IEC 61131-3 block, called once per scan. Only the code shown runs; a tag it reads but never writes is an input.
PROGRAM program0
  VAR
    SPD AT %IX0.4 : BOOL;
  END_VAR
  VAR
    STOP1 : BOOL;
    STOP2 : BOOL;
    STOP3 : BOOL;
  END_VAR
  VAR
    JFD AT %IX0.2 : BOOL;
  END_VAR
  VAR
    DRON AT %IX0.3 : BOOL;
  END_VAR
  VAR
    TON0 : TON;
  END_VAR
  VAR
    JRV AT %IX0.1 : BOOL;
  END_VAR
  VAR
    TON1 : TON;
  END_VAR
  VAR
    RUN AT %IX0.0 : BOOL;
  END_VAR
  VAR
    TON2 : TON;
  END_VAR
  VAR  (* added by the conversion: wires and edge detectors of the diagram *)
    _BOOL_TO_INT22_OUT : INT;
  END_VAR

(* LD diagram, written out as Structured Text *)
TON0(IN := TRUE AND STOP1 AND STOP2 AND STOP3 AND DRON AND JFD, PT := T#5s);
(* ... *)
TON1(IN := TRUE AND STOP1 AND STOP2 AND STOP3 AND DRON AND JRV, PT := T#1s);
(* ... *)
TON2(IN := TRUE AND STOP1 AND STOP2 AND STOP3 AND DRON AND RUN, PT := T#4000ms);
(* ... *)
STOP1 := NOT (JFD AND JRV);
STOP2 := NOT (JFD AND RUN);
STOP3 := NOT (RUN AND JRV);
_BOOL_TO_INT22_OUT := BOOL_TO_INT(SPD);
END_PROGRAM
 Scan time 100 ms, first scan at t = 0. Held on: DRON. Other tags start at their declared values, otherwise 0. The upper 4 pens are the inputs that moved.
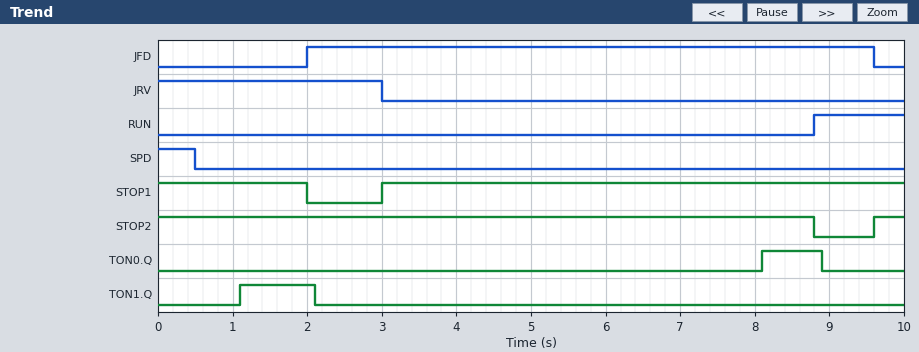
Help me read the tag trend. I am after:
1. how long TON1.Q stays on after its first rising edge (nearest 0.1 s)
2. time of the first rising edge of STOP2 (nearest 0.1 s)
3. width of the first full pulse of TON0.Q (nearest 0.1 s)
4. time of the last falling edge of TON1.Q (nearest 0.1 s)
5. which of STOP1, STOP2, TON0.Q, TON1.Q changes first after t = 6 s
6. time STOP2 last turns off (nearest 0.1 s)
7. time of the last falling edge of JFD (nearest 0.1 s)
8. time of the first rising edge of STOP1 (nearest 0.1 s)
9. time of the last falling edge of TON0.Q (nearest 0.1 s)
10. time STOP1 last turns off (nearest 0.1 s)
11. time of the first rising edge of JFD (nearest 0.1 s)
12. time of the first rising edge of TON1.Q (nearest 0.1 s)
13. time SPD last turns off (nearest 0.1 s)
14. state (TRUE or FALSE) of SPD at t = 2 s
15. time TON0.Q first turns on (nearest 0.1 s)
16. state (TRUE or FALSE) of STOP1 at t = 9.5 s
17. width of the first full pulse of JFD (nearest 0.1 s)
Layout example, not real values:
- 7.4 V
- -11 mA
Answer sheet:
- 1.0 s
- 9.6 s
- 0.8 s
- 2.1 s
- TON0.Q
- 8.8 s
- 9.6 s
- 3.0 s
- 8.9 s
- 2.0 s
- 2.0 s
- 1.1 s
- 0.5 s
- FALSE
- 8.1 s
- TRUE
- 7.6 s
